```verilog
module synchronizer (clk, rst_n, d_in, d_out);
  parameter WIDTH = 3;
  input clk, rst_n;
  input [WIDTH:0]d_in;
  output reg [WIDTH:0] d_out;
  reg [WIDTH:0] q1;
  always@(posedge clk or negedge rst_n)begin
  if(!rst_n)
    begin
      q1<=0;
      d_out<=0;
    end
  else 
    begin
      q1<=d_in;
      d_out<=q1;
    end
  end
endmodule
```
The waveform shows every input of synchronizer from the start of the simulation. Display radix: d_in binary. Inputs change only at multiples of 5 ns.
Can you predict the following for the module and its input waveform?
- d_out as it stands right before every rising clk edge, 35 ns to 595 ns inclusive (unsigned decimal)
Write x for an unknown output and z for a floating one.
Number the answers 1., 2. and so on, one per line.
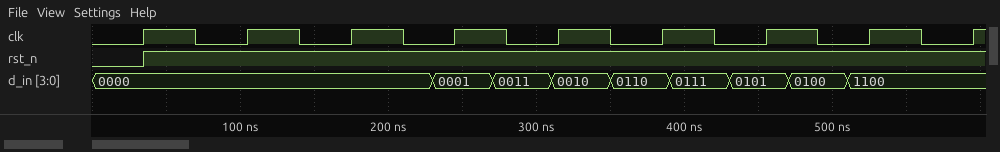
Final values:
1. 0, 0, 0, 0, 0, 1, 2, 6, 5
